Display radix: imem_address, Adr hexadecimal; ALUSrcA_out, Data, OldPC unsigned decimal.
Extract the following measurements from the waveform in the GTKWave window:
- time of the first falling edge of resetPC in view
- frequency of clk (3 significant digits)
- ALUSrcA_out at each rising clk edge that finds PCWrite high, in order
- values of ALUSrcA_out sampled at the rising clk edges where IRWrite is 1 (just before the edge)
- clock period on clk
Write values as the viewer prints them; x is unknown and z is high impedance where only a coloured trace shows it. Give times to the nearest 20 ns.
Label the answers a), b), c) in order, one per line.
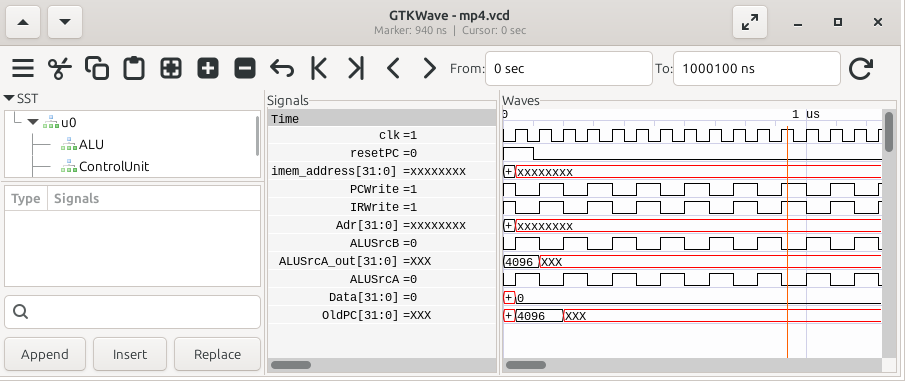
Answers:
a) 100 ns
b) 12.5 MHz
c) 4096, XXX, XXX, XXX, XXX, XXX, XXX, XXX
d) 4096, XXX, XXX, XXX, XXX, XXX, XXX, XXX
e) 80 ns
